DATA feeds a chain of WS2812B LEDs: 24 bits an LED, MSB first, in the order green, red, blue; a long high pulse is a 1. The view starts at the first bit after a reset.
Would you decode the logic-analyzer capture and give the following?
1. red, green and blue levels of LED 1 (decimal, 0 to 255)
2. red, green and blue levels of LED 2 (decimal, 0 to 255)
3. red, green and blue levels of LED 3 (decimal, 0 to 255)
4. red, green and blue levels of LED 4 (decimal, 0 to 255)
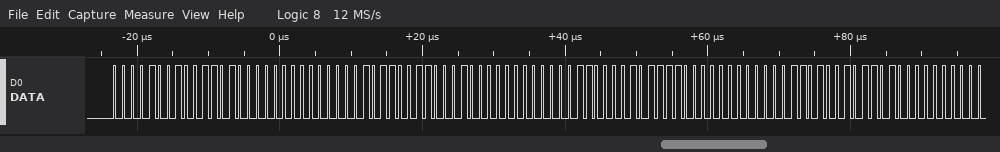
52, 9, 0
49, 11, 0
47, 12, 0
45, 13, 0
